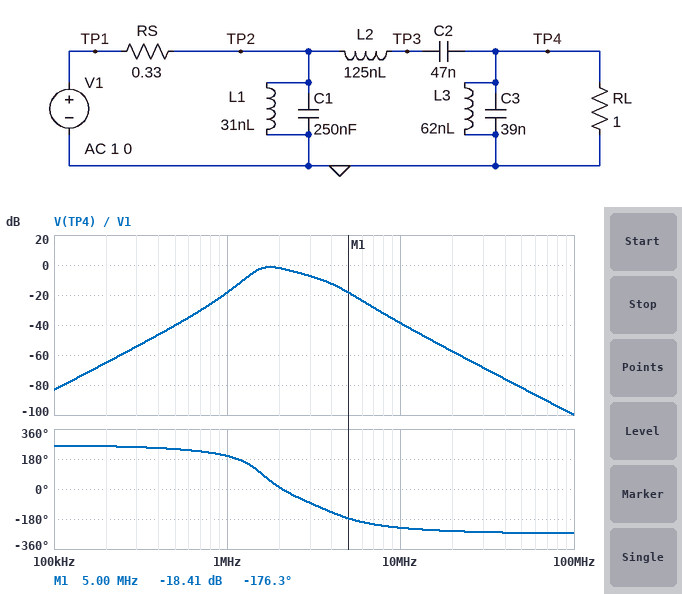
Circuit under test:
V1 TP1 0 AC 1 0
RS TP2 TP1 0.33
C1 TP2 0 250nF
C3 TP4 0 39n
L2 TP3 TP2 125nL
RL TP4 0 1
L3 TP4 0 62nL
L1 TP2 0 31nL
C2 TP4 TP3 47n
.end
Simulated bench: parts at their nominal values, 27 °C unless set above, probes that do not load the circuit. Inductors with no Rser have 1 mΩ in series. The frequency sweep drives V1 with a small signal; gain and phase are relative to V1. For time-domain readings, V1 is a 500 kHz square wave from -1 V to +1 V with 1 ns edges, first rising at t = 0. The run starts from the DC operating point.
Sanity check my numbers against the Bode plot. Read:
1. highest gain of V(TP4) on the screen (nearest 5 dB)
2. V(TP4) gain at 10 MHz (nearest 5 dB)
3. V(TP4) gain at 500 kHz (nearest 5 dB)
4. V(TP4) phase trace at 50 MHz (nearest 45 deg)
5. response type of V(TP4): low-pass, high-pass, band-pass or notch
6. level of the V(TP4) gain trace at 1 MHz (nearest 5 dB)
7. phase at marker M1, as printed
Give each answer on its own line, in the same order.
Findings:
0 dB
-40 dB
-40 dB
-270 deg
band-pass
-20 dB
-176.3 deg
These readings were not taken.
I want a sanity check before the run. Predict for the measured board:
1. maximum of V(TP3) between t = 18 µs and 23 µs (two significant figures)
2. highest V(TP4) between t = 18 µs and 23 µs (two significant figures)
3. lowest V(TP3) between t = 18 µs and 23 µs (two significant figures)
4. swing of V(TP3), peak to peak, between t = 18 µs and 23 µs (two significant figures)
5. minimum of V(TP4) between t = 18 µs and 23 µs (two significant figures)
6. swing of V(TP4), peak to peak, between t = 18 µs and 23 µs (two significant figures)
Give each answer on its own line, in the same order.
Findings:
1.6 V
470 mV
-1.6 V
3.1 V
-470 mV
950 mV
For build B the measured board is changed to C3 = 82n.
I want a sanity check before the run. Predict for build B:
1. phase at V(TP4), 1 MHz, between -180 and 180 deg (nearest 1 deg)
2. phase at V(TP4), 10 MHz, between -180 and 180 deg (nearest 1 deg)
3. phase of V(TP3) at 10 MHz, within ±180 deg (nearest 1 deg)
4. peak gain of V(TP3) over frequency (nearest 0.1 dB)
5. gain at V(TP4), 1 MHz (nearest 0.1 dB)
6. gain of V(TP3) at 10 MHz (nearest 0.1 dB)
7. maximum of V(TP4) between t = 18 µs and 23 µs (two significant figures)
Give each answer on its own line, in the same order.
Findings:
-166 deg
113 deg
106 deg
5.2 dB
-17.3 dB
-36.8 dB
540 mV
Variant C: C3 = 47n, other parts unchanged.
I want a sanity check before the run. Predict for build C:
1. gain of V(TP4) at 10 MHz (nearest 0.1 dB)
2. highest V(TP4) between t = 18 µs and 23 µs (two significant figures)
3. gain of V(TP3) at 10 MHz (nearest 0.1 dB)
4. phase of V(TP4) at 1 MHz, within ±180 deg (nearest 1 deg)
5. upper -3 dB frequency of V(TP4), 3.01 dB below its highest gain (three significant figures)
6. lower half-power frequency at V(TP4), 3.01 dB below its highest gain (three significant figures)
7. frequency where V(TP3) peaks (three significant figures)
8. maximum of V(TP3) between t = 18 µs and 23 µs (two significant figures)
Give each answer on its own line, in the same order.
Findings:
-40.4 dB
490 mV
-34.6 dB
-163 deg
2.50 MHz
1.43 MHz
1.54 MHz
1.6 V
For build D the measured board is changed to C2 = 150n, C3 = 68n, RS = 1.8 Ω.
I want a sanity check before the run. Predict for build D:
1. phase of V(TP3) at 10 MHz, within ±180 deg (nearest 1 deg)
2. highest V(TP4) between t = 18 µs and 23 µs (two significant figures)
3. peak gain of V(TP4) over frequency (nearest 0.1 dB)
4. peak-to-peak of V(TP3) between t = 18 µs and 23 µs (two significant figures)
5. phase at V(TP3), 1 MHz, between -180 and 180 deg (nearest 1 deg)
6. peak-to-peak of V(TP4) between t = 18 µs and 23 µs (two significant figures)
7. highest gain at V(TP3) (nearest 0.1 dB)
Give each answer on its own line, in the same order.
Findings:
102 deg
120 mV
-9.0 dB
390 mV
-54 deg
250 mV
-3.2 dB
